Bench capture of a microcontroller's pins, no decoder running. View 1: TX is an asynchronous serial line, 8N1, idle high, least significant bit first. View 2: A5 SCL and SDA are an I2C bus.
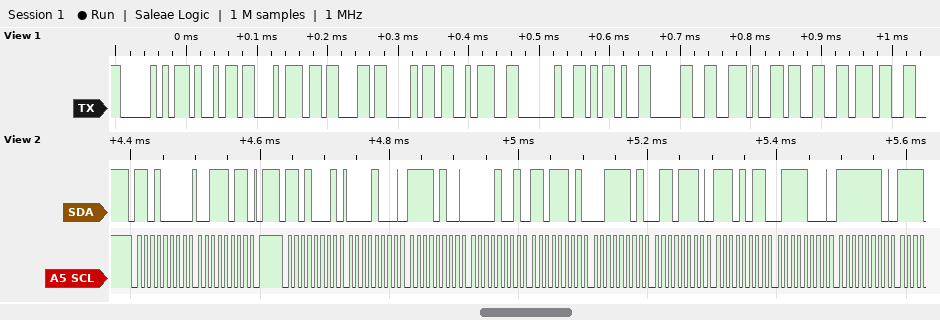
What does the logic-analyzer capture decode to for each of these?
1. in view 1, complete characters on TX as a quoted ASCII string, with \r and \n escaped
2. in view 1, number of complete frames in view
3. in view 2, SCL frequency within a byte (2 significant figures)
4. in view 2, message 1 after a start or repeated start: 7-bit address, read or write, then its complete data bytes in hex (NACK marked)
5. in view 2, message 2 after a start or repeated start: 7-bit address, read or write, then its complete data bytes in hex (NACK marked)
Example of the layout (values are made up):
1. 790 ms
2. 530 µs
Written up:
1. "Pitch: -0.37"
2. 12
3. 100 kHz
4. 0x68 write: 3B
5. 0x68 read: 08 F4 09 DD 3D 6E EB 78 FE
